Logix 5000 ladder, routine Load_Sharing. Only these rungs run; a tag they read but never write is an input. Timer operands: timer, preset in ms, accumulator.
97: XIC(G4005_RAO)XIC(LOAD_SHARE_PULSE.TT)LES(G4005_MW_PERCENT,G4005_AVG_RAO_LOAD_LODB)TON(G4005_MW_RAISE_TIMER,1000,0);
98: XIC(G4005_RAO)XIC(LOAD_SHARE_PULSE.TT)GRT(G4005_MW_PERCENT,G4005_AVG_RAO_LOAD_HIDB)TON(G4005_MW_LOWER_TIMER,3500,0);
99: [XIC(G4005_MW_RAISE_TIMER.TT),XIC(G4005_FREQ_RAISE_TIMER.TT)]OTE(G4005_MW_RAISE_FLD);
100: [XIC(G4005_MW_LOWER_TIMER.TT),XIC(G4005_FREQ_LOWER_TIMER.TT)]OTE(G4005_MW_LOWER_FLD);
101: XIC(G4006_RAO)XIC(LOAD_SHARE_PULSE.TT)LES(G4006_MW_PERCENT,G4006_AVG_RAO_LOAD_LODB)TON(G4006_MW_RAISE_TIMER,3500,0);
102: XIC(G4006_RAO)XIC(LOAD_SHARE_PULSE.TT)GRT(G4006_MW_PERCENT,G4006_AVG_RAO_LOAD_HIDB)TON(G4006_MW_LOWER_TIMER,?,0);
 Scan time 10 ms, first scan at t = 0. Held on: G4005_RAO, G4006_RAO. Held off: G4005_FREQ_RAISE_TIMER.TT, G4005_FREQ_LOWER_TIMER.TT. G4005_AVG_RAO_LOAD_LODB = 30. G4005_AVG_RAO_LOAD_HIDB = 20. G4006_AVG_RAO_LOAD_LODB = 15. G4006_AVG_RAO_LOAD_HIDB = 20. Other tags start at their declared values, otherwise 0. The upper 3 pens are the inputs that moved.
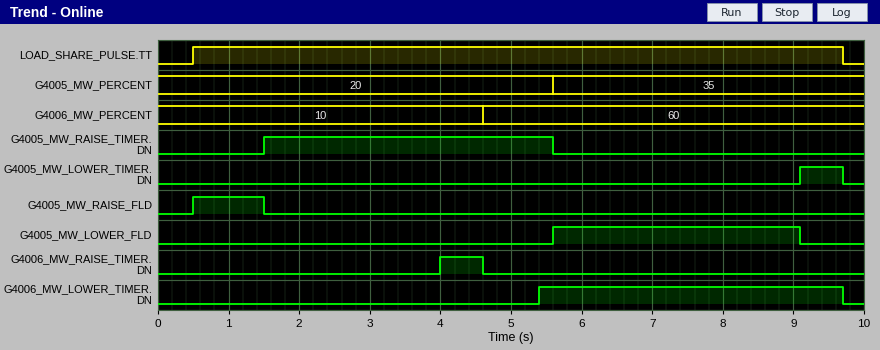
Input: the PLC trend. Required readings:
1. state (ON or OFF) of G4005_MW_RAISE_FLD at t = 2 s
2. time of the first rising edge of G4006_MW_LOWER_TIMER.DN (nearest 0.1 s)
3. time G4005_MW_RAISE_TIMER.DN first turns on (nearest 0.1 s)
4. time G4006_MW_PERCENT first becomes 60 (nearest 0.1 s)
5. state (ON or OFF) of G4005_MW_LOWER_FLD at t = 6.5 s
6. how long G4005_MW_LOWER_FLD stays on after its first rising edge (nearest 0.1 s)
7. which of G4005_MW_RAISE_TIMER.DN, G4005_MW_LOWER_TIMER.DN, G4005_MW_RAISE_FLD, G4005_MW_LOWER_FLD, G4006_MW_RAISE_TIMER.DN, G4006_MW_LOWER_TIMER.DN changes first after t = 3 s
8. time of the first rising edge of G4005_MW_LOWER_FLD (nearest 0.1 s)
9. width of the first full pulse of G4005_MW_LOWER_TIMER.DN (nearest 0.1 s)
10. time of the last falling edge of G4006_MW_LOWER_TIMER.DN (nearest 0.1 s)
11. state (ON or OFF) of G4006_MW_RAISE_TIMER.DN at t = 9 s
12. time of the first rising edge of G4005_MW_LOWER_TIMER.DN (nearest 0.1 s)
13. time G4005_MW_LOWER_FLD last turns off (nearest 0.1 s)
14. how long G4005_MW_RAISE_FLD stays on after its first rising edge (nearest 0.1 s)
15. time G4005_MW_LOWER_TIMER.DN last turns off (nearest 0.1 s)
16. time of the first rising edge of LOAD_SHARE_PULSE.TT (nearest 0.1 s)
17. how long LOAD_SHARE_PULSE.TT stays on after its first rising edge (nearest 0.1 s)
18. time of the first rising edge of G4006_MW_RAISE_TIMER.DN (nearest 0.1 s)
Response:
OFF
5.4 s
1.5 s
4.6 s
ON
3.5 s
G4006_MW_RAISE_TIMER.DN
5.6 s
0.6 s
9.7 s
OFF
9.1 s
9.1 s
1.0 s
9.7 s
0.5 s
9.2 s
4.0 s
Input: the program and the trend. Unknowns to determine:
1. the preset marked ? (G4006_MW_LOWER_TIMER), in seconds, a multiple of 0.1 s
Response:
0.8 s
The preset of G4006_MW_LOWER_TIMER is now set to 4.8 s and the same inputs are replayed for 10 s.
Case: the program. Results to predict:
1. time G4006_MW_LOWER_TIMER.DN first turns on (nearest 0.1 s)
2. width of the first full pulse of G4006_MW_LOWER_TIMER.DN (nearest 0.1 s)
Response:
9.4 s
0.3 s
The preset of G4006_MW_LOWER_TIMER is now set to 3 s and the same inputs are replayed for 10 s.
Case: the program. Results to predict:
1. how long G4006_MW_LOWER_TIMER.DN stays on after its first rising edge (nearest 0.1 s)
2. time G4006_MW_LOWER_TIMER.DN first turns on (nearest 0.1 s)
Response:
2.1 s
7.6 s
